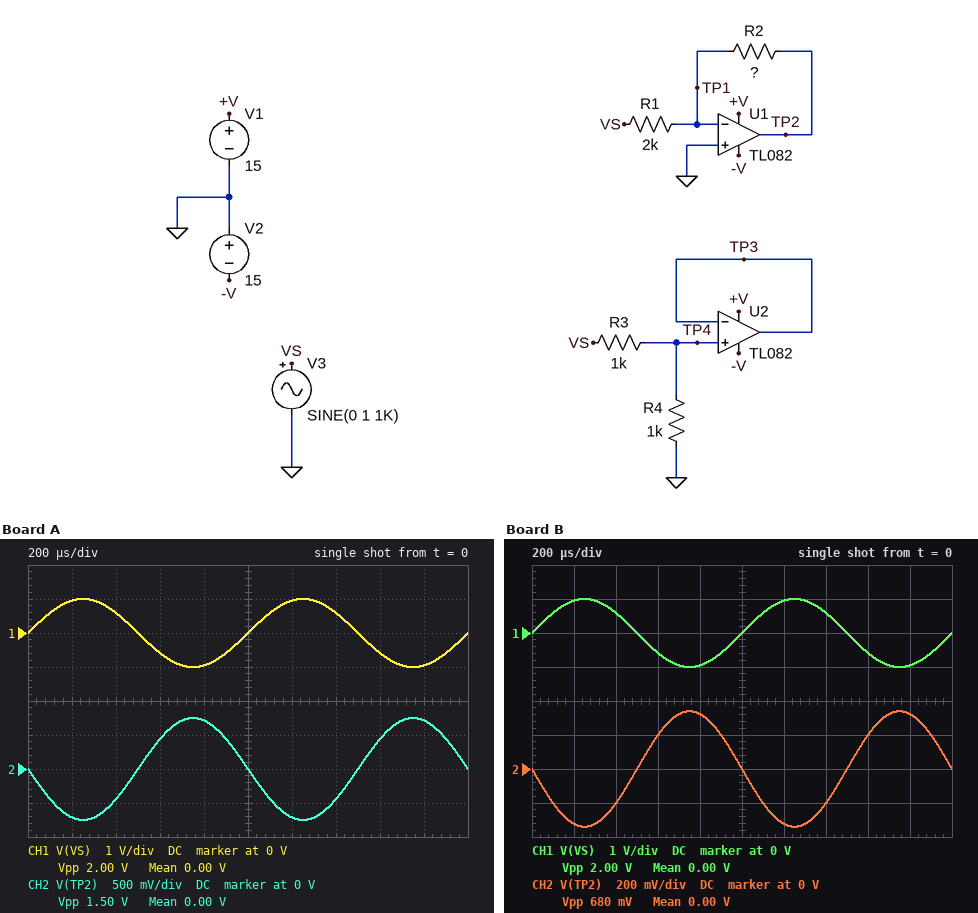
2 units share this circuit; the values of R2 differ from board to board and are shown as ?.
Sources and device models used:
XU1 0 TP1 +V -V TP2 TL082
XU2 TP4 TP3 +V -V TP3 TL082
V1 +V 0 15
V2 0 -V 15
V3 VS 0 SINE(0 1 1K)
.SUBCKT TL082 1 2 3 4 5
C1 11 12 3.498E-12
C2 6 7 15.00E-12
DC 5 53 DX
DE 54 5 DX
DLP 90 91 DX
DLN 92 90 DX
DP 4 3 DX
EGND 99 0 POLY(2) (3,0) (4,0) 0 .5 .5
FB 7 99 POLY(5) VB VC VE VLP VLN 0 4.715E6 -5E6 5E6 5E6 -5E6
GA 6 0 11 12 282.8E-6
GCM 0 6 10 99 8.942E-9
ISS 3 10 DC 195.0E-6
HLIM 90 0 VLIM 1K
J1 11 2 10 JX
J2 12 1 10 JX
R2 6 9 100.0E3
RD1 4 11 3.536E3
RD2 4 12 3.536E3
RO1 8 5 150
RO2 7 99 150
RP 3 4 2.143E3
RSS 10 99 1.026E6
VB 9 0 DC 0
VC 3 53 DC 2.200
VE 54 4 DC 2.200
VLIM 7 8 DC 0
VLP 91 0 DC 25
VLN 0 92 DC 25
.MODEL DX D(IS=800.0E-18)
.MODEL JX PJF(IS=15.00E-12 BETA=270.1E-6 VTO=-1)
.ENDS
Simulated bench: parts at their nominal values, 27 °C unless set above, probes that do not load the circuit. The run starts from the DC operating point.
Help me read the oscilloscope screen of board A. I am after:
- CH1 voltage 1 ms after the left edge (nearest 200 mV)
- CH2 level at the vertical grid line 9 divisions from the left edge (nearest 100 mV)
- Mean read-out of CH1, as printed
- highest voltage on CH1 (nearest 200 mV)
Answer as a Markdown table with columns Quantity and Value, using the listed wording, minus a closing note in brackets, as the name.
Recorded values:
| Quantity | Value |
|---|---|
| CH1 voltage 1 ms after the left edge | 0 V |
| CH2 level at the vertical grid line 9 divisions from the left edge | 700 mV |
| Mean read-out of CH1, as printed | 0.00 V |
| highest voltage on CH1 | 1.0 V |
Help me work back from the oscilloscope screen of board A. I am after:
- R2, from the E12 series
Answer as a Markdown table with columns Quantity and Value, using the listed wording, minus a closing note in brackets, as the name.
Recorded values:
| Quantity | Value |
|---|---|
| R2, from the E12 series | 1.5 kΩ |
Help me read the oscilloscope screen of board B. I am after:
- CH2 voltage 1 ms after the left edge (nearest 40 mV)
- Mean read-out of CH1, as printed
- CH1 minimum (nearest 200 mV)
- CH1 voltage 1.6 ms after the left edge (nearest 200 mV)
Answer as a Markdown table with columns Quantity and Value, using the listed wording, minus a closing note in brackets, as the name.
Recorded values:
| Quantity | Value |
|---|---|
| CH2 voltage 1 ms after the left edge | 0 V |
| Mean read-out of CH1, as printed | 0.00 V |
| CH1 minimum | -1.0 V |
| CH1 voltage 1.6 ms after the left edge | -600 mV |
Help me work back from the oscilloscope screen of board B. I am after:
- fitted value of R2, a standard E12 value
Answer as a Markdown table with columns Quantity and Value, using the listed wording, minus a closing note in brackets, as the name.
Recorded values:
| Quantity | Value |
|---|---|
| fitted value of R2, a standard E12 value | 680 Ω |
